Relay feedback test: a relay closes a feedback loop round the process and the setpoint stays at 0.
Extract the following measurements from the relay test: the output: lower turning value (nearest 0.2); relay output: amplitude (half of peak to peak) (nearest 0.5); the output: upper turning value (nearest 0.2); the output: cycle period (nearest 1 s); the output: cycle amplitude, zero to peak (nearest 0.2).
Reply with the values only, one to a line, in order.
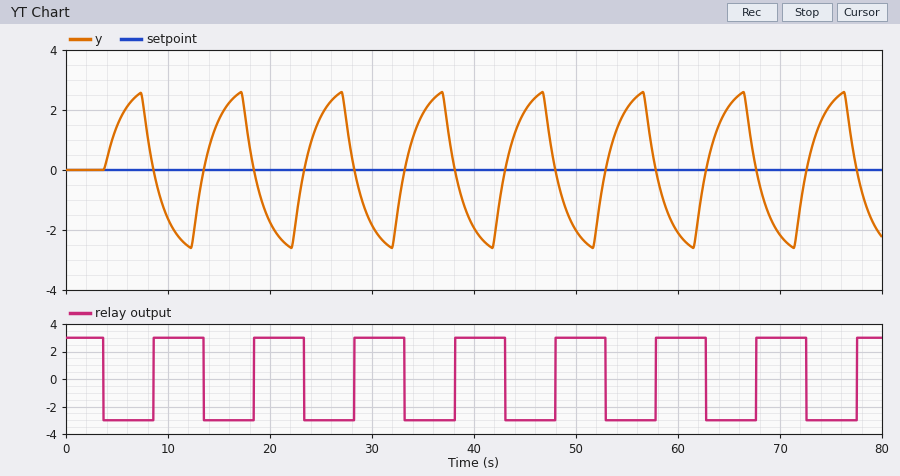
-2.6
3.0
2.6
10 s
2.6
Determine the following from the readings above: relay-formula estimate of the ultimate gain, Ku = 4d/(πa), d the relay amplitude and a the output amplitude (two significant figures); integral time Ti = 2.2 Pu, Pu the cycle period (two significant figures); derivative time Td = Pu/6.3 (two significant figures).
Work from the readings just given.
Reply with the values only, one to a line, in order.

1.5
22 s
1.6 s
